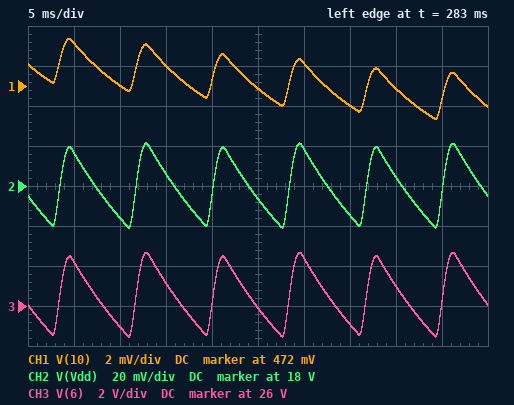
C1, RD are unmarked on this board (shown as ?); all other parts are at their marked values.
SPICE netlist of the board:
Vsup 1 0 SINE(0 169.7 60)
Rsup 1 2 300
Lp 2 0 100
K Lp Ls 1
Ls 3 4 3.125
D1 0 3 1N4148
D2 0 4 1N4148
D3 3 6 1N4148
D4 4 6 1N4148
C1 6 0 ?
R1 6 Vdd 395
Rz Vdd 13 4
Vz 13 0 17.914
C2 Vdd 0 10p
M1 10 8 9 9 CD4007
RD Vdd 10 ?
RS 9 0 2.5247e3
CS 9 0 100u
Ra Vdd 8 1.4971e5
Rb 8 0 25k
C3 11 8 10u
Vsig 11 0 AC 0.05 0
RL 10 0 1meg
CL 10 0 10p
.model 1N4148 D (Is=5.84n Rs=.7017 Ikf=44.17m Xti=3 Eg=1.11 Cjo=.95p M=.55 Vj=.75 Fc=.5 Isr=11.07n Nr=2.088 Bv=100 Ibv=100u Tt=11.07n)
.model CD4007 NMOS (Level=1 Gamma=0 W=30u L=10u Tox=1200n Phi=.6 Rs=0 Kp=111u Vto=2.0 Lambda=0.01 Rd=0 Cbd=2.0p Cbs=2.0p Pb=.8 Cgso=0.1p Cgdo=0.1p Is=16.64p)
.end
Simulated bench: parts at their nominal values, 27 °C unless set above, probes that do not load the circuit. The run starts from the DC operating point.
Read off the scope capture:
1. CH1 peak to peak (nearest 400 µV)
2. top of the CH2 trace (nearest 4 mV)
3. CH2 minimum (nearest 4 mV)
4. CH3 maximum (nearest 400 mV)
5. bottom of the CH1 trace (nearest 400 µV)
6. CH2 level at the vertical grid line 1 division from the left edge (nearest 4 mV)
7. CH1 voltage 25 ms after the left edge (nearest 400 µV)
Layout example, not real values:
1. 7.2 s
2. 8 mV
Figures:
1. 4.0 mV
2. 18.020 V
3. 17.980 V
4. 28.8 V
5. 470.4 mV
6. 18.016 V
7. 472.0 mV
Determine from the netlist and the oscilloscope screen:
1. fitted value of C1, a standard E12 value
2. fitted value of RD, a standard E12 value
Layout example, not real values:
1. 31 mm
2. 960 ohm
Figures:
1. 33 µF
2. 470 kΩ
